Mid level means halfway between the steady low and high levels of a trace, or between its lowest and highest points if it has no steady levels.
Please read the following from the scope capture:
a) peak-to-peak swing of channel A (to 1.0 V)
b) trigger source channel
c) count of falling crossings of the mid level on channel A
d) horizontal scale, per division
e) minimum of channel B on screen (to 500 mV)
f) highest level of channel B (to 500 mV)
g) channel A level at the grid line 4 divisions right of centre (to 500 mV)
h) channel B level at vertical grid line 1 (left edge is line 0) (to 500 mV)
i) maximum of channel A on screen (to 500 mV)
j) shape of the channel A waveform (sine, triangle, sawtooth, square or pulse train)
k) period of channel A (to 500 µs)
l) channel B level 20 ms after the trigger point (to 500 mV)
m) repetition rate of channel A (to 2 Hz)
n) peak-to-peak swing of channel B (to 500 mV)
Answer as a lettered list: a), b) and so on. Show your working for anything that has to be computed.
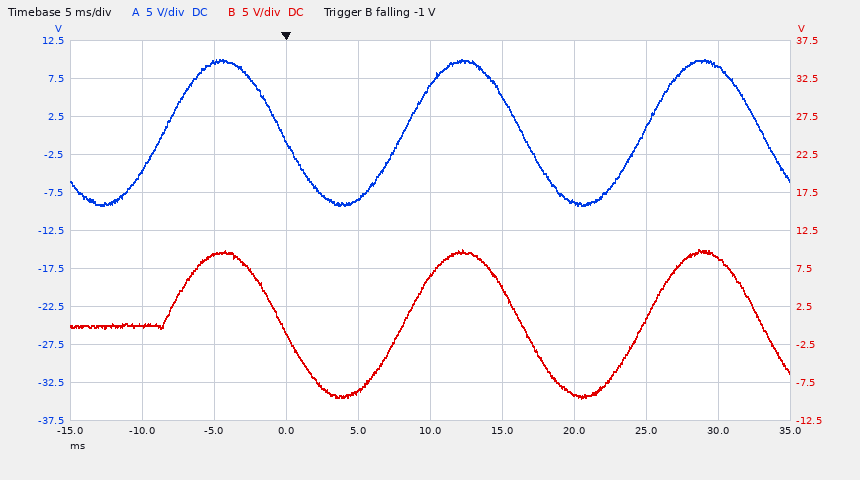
a) 19.0 V
b) channel B
c) 3
d) 5 ms
e) -9.5 V
f) 10.0 V
g) 9.0 V
h) 0.0 V
i) 10.0 V
j) sine
k) 16.5 ms
l) -9.0 V
m) 1 / 16.5 ms ≈ 60.6 Hz, so 60 Hz to the nearest 2 Hz
n) 10.0 V − (-9.5 V) = 19.5 V
